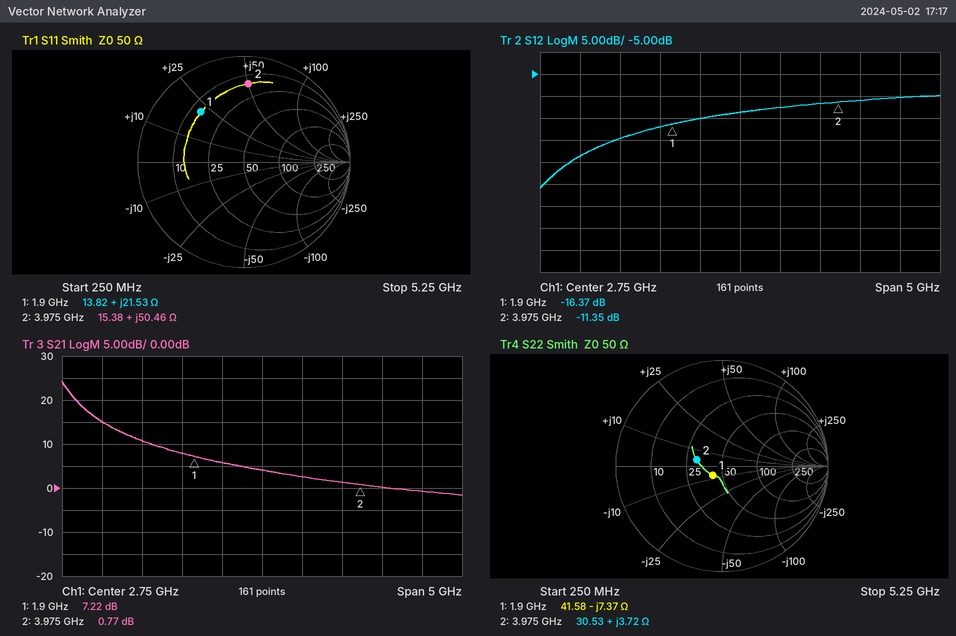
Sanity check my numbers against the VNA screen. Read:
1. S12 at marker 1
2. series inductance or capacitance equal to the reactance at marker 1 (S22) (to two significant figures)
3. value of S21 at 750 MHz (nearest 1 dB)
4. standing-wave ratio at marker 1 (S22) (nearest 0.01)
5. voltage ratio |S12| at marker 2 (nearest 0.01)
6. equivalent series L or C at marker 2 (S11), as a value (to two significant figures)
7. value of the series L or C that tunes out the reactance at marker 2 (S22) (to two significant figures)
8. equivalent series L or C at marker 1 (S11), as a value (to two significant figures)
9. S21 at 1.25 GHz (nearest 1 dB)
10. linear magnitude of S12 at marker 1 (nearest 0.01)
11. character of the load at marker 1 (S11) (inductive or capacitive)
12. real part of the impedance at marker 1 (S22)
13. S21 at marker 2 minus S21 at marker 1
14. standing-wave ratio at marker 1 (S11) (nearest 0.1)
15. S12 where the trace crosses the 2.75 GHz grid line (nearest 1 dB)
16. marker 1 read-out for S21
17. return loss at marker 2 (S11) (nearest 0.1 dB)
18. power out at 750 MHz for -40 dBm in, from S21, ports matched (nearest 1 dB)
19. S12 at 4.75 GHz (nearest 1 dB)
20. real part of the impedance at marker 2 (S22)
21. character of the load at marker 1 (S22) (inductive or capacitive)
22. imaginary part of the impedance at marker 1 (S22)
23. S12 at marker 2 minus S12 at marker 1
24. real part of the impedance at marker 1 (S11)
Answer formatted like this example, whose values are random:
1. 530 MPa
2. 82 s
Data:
1. -16.37 dB
2. 11 pF
3. 15 dB
4. 1.28
5. 0.27
6. 2.0 nH
7. 11 pF
8. 1.8 nH
9. 11 dB
10. 0.15
11. inductive
12. 41.58 Ω
13. -6.45 dB
14. 4.3
15. -14 dB
16. 7.22 dB
17. 2.6 dB
18. -25 dBm
19. -10 dB
20. 30.53 Ω
21. capacitive
22. -7.37 Ω
23. 5.02 dB
24. 13.82 Ω
